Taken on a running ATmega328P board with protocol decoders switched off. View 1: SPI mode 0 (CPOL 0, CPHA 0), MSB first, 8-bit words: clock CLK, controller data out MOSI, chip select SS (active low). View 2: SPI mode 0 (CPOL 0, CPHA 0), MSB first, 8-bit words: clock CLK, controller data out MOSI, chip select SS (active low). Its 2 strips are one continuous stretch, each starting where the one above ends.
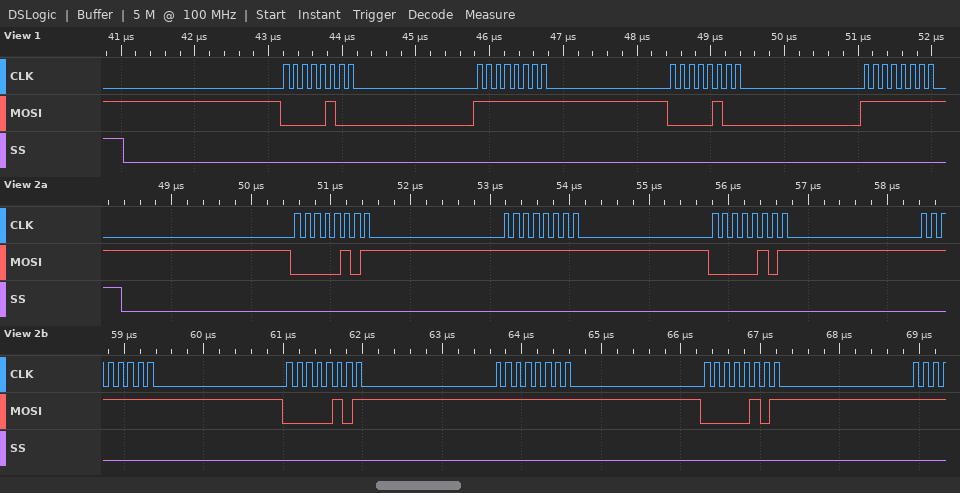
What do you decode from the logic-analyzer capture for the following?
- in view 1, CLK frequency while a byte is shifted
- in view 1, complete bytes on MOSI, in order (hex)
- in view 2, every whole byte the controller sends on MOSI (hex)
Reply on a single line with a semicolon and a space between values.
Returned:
8 MHz; 04 FF 04 FF; 05 FF 05 FF 05 FF 05
